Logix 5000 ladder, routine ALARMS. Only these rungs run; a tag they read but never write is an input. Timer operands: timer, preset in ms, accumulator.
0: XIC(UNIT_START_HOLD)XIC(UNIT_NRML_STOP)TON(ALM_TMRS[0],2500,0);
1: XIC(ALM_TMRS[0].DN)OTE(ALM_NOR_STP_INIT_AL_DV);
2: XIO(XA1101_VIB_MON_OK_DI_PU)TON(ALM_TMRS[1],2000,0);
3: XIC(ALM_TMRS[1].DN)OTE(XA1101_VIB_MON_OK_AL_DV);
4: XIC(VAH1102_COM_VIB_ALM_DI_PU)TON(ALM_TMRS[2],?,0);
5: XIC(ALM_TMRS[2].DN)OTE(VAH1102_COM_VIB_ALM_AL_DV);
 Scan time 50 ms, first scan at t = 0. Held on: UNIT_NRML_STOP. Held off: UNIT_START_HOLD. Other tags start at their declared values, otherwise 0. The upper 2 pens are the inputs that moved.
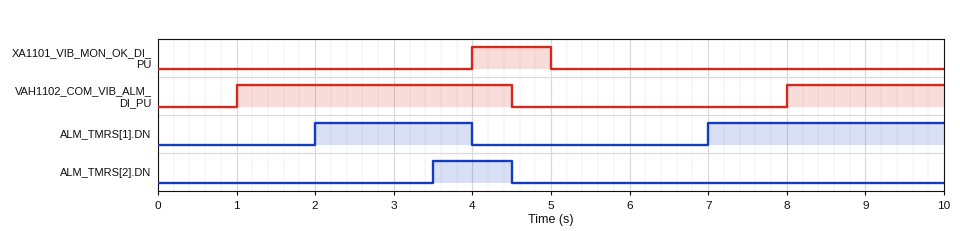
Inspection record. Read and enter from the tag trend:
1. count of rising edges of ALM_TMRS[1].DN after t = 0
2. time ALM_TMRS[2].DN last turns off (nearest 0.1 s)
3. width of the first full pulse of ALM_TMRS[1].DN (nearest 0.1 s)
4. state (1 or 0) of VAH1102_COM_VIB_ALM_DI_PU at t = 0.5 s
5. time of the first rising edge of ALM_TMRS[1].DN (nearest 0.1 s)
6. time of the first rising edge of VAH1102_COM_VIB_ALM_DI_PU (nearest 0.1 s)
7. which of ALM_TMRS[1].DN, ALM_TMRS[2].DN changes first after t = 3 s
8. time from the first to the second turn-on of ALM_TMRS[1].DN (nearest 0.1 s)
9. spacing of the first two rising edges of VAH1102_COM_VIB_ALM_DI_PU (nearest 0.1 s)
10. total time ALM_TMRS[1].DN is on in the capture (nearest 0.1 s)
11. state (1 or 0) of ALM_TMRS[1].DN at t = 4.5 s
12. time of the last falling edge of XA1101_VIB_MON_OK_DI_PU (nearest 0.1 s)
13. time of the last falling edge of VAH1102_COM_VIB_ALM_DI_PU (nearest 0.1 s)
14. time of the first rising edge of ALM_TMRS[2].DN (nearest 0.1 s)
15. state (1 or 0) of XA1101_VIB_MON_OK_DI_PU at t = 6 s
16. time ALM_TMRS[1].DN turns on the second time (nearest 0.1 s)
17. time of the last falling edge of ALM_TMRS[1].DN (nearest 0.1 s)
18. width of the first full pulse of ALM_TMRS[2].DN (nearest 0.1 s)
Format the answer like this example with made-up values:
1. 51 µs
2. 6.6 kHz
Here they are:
1. 2
2. 4.5 s
3. 2.0 s
4. 0
5. 2.0 s
6. 1.0 s
7. ALM_TMRS[2].DN
8. 5.0 s
9. 7.0 s
10. 5.0 s
11. 0
12. 5.0 s
13. 4.5 s
14. 3.5 s
15. 0
16. 7.0 s
17. 4.0 s
18. 1.0 s
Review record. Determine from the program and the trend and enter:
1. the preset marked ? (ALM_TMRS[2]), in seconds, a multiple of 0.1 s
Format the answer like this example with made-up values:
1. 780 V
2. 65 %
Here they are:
1. 2.5 s
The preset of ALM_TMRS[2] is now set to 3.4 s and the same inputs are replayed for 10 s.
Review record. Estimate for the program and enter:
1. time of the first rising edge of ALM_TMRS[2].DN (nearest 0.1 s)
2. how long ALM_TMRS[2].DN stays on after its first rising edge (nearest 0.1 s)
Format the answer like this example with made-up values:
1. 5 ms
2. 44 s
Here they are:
1. 4.4 s
2. 0.1 s
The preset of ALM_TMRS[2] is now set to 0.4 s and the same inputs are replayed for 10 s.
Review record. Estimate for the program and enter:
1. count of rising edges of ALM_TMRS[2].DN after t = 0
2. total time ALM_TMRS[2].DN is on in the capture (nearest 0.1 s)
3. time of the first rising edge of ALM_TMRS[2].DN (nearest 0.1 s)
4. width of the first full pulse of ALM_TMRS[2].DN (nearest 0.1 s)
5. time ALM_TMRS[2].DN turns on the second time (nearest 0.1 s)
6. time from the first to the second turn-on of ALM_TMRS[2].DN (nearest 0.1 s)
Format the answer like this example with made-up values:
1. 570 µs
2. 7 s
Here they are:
1. 2
2. 4.7 s
3. 1.4 s
4. 3.1 s
5. 8.4 s
6. 7.0 s
